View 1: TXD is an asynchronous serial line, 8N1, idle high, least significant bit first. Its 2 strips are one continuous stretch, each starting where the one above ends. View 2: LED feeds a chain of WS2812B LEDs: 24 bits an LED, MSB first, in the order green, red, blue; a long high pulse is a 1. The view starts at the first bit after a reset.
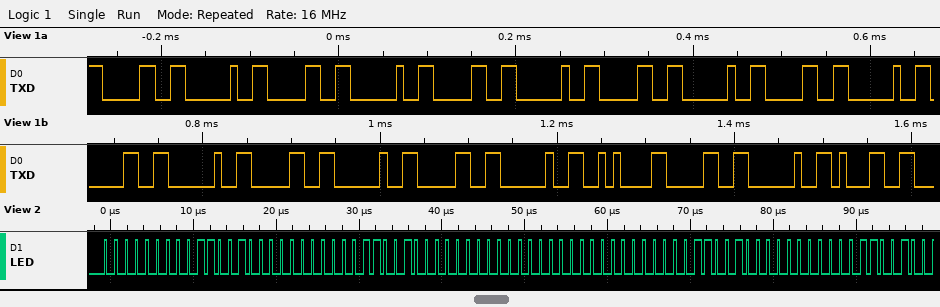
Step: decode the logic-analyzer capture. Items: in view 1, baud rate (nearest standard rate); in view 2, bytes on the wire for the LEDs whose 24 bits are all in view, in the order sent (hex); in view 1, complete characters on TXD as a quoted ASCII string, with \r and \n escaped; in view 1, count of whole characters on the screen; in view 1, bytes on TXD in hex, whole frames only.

115200 baud
00 64 00 64 00 00 00 64 00
"0 0 0 0 0 0 0 0 \n0 1"
20
30 20 30 20 30 20 30 20 30 20 30 20 30 20 30 20 0A 30 20 31
